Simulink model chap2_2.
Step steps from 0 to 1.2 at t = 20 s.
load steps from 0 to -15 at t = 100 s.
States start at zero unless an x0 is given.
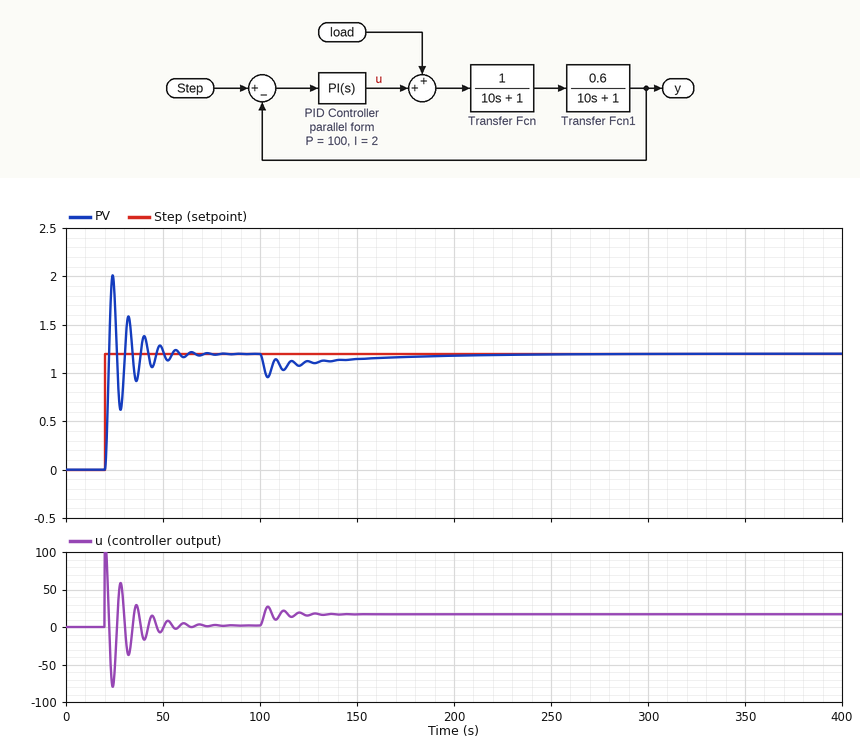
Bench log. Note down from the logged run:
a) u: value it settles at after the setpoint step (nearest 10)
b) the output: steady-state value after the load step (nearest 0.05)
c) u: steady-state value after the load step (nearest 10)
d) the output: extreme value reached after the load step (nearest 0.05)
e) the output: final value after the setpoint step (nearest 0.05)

0
1.20
20
0.95
1.20
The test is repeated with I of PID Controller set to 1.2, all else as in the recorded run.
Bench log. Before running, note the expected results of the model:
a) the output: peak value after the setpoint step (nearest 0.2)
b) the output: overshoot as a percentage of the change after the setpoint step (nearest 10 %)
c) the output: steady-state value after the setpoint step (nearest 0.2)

2.0
70 %
1.2
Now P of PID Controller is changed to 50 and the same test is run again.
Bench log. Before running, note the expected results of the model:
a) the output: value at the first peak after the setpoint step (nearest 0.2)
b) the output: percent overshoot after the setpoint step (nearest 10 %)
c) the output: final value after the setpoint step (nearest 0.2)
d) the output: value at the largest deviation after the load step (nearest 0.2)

2.0
60 %
1.2
0.8
